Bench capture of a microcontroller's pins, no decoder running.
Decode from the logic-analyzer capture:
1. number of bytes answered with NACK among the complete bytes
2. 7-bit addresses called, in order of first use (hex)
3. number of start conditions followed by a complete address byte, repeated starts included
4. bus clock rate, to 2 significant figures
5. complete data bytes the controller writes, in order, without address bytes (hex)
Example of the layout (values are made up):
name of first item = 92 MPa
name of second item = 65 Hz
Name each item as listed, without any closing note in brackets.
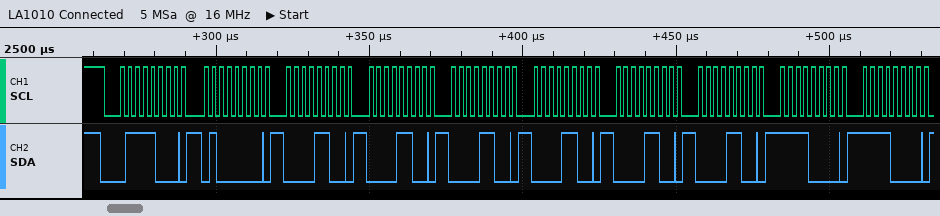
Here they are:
number of bytes answered with NACK among the complete bytes = 0
7-bit addresses called, in order of first use = 0x3C
number of start conditions followed by a complete address byte, repeated starts included = 1
bus clock rate, to 2 significant figures = 400 kHz
complete data bytes the controller writes, in order, without address bytes = 40 0C 0C 0C 0C 0C 0C F0 F0
